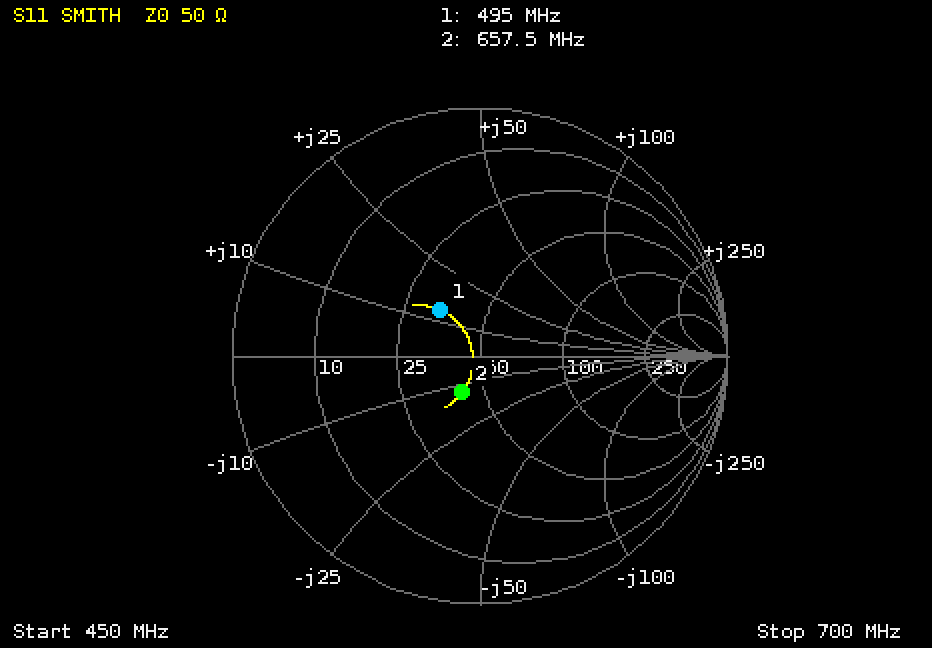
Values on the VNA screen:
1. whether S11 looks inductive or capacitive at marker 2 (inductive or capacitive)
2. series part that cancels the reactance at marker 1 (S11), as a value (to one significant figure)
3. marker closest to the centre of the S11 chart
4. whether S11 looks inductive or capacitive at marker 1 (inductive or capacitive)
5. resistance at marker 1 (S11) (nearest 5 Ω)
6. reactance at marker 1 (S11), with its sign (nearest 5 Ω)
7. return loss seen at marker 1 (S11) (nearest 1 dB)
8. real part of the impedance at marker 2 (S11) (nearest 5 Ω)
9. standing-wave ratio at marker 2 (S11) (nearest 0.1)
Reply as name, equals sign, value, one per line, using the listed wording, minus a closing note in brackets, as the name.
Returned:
whether S11 looks inductive or capacitive at marker 2 = capacitive
series part that cancels the reactance at marker 1 (S11), as a value = 20 pF
marker closest to the centre of the S11 chart = marker 2
whether S11 looks inductive or capacitive at marker 1 = inductive
resistance at marker 1 (S11) = 35 Ω
reactance at marker 1 (S11), with its sign = +15 Ω
return loss seen at marker 1 (S11) = 12 dB
real part of the impedance at marker 2 (S11) = 40 Ω
standing-wave ratio at marker 2 (S11) = 1.4
